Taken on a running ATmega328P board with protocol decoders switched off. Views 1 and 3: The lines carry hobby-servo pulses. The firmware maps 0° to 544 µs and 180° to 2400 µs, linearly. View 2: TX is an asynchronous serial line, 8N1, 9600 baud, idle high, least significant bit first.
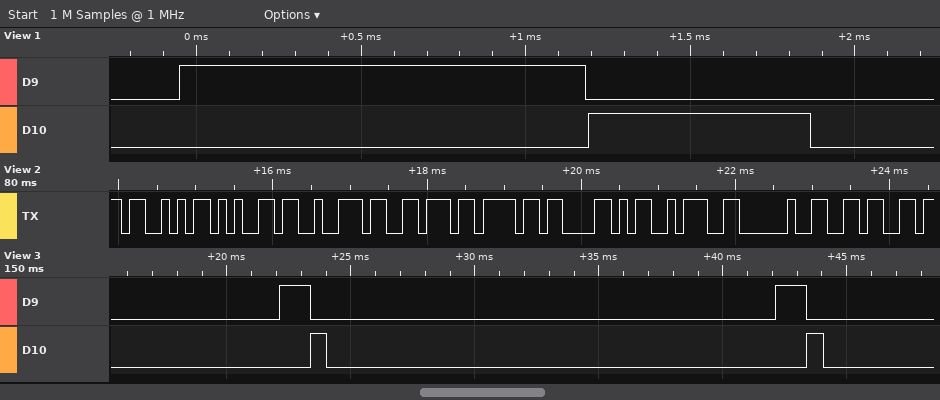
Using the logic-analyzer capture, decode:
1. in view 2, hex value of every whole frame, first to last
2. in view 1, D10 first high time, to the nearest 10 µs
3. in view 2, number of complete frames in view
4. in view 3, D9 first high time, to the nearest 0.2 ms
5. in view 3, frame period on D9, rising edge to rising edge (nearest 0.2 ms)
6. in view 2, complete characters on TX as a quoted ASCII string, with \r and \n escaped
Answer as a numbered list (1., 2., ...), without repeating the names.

1. 53 65 72 76 6F 58 3A 20 36
2. 670 µs
3. 9
4. 1.2 ms
5. 20.0 ms
6. "ServoX: 6"
